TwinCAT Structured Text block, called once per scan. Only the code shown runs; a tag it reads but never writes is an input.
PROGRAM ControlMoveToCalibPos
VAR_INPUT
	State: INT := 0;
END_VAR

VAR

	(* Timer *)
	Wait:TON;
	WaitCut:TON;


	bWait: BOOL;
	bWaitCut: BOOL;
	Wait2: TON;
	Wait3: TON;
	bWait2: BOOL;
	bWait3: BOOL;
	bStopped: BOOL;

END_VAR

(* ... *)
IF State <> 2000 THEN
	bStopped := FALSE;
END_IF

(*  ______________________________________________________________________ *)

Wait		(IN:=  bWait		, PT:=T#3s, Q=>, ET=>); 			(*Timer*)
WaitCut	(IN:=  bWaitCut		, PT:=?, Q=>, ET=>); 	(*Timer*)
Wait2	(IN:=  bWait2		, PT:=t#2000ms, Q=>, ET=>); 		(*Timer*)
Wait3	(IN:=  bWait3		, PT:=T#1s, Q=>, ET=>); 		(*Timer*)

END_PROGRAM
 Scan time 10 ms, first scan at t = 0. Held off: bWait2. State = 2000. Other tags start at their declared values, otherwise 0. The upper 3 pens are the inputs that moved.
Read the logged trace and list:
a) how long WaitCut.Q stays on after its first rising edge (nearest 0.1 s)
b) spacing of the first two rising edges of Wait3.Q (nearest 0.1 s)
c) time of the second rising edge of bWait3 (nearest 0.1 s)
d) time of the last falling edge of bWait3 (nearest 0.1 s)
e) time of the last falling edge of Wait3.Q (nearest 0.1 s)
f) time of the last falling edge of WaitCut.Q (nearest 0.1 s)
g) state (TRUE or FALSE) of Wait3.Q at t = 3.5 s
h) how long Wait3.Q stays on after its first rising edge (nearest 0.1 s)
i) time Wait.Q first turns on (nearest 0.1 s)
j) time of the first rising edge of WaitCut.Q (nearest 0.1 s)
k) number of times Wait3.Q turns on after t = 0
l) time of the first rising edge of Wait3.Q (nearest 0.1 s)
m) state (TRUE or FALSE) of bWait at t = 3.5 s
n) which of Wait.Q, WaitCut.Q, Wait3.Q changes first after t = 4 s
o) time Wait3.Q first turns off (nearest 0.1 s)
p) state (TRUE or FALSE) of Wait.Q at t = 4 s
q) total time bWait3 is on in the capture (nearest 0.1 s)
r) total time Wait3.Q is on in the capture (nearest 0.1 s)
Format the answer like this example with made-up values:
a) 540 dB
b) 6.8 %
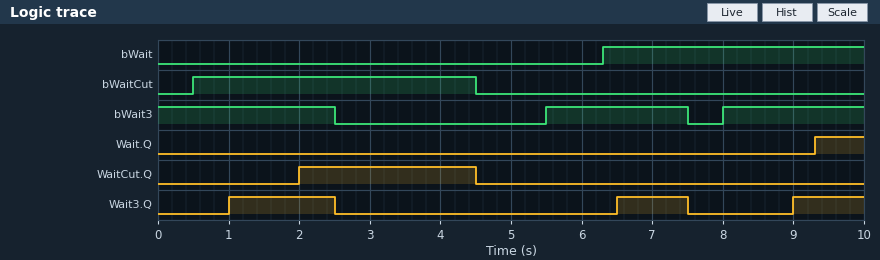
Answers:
a) 2.5 s
b) 5.5 s
c) 8.0 s
d) 7.5 s
e) 7.5 s
f) 4.5 s
g) FALSE
h) 1.5 s
i) 9.3 s
j) 2.0 s
k) 3
l) 1.0 s
m) FALSE
n) WaitCut.Q
o) 2.5 s
p) FALSE
q) 6.5 s
r) 3.5 s
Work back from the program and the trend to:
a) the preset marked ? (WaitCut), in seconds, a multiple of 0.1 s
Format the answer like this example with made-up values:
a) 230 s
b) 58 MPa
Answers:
a) 1.5 s
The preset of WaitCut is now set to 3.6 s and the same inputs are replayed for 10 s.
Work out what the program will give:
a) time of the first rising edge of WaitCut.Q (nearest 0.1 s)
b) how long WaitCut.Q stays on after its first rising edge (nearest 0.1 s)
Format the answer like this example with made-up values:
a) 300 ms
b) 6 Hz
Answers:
a) 4.1 s
b) 0.4 s
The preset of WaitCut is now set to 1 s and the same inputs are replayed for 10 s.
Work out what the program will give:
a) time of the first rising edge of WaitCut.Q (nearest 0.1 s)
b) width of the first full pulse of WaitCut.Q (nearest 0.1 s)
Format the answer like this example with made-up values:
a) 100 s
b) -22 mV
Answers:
a) 1.5 s
b) 3.0 s
